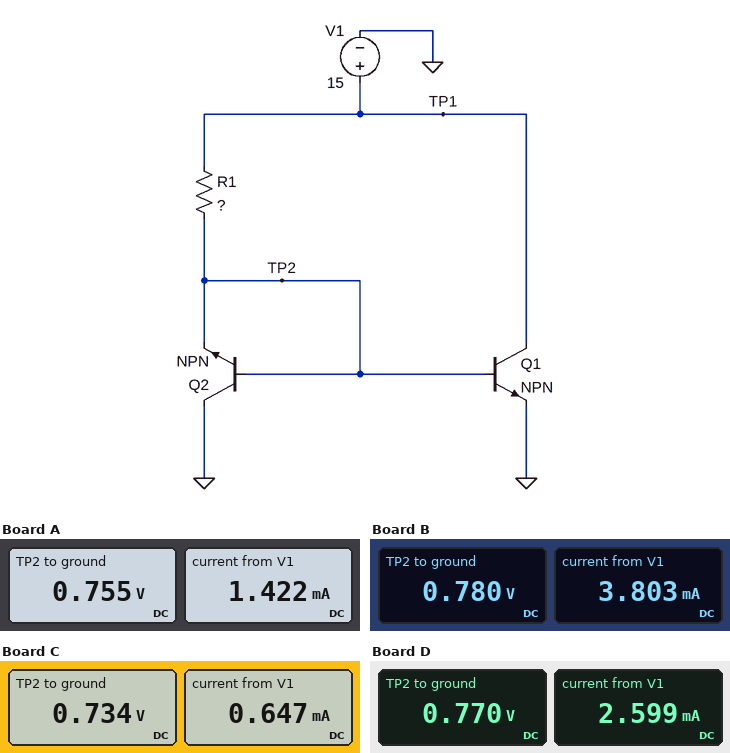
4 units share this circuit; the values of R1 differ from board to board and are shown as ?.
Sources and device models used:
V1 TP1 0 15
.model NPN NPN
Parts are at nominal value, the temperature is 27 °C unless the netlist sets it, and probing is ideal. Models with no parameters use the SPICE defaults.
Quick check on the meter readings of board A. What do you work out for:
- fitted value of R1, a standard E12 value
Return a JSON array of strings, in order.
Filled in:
["15 kΩ"]
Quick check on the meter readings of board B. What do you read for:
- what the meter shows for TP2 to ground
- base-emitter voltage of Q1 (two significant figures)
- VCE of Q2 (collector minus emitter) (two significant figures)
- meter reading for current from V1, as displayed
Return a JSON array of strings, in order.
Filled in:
["0.780 V", "780 mV", "-780 mV", "3.803 mA"]
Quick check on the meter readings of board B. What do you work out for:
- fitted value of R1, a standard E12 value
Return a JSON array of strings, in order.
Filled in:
["5.6 kΩ"]
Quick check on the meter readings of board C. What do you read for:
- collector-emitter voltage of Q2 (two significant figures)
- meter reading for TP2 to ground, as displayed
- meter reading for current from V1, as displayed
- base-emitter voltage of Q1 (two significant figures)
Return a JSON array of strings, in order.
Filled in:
["-730 mV", "0.734 V", "0.647 mA", "730 mV"]
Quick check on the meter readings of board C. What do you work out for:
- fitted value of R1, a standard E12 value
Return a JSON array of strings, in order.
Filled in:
["33 kΩ"]
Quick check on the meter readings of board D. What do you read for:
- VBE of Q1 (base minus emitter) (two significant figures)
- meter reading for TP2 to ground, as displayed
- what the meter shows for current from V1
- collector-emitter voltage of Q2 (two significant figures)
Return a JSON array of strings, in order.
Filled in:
["770 mV", "0.770 V", "2.599 mA", "-770 mV"]
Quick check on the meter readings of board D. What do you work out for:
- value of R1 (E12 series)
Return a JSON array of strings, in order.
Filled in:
["8.2 kΩ"]
